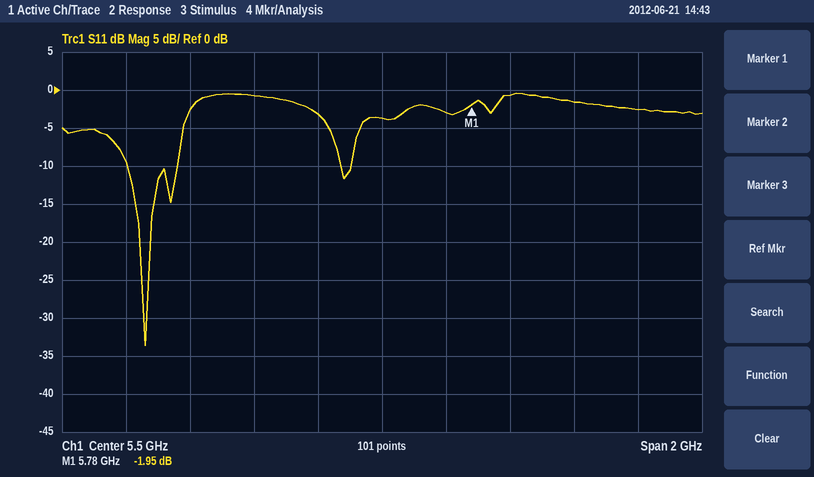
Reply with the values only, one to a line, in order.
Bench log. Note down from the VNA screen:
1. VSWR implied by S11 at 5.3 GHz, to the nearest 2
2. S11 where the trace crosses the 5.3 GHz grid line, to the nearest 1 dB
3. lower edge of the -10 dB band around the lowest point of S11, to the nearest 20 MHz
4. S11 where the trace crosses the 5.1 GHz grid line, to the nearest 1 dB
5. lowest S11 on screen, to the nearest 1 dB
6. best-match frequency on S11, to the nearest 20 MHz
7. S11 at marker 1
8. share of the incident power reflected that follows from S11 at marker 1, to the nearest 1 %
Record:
6
-3 dB
4.70 GHz
-1 dB
-34 dB
4.76 GHz
-1.95 dB
64 %
